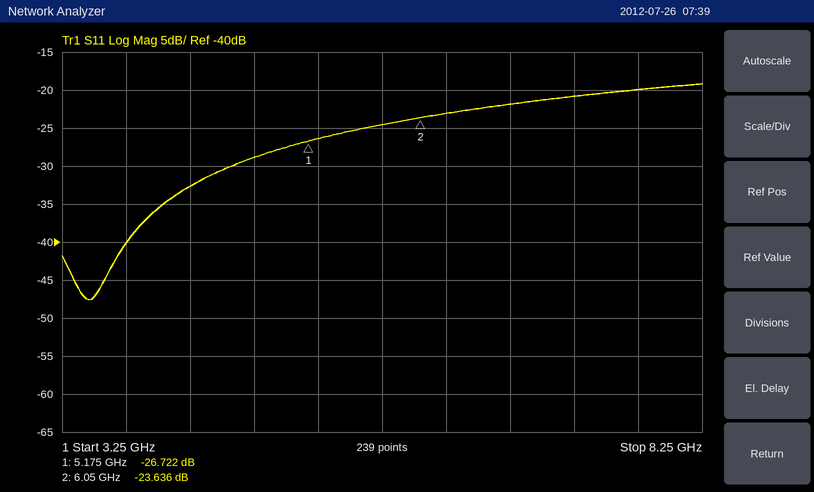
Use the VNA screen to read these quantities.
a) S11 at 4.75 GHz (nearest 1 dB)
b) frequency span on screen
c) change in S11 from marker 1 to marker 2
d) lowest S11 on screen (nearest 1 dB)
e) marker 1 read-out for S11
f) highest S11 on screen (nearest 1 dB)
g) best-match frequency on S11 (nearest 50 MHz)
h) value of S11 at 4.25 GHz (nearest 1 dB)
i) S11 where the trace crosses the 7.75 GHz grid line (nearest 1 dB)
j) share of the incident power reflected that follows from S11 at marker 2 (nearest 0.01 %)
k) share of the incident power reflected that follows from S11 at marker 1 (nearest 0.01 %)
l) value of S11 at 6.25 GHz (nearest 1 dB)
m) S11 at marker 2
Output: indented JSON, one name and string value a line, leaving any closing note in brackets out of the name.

{
  "S11 at 4.75 GHz": "-29 dB",
  "frequency span on screen": "5 GHz",
  "change in S11 from marker 1 to marker 2": "3.086 dB",
  "lowest S11 on screen": "-48 dB",
  "marker 1 read-out for S11": "-26.722 dB",
  "highest S11 on screen": "-19 dB",
  "best-match frequency on S11": "3.45 GHz",
  "value of S11 at 4.25 GHz": "-33 dB",
  "S11 where the trace crosses the 7.75 GHz grid line": "-20 dB",
  "share of the incident power reflected that follows from S11 at marker 2": "0.43 %",
  "share of the incident power reflected that follows from S11 at marker 1": "0.21 %",
  "value of S11 at 6.25 GHz": "-23 dB",
  "S11 at marker 2": "-23.636 dB"
}
